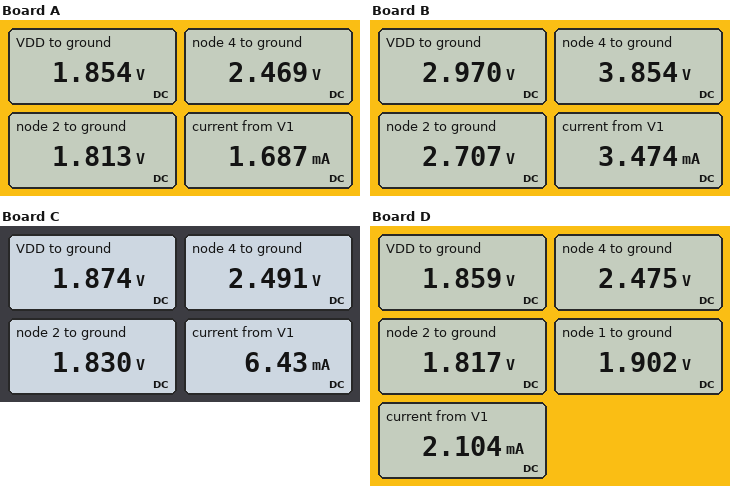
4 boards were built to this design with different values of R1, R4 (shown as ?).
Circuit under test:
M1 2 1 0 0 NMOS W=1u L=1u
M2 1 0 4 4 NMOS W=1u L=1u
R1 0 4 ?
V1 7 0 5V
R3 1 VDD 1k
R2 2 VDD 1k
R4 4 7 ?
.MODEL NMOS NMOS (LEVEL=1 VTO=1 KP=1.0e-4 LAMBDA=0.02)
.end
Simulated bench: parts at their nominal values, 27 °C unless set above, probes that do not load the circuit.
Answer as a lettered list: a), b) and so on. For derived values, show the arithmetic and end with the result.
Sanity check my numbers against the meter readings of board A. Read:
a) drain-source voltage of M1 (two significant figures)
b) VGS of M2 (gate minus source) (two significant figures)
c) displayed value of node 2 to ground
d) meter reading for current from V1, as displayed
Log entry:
a) 1.813 V = 1.8 V
b) 0 V - 2.469 V = -2.5 V
c) 1.813 V
d) 1.687 mA
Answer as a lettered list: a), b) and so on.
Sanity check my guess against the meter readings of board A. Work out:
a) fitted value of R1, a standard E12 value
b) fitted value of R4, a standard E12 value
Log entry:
a) 1.5 kΩ
b) 1.5 kΩ
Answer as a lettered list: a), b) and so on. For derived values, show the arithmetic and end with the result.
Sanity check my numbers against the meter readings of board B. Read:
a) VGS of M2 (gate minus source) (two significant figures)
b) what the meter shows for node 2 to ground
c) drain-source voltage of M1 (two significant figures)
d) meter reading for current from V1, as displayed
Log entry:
a) 0 V - 3.854 V = -3.9 V
b) 2.707 V
c) 2.707 V = 2.7 V
d) 3.474 mA
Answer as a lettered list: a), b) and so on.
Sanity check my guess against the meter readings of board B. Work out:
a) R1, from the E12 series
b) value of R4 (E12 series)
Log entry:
a) 1.2 kΩ
b) 330 Ω
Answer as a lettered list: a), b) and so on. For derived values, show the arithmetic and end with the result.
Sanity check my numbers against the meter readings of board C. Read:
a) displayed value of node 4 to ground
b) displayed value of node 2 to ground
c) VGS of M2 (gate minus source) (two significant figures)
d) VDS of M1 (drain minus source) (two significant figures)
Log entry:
a) 2.491 V
b) 1.830 V
c) 0 V - 2.491 V = -2.5 V
d) 1.83 V = 1.8 V
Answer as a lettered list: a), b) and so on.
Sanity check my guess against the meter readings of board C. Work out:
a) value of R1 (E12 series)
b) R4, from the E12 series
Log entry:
a) 390 Ω
b) 390 Ω
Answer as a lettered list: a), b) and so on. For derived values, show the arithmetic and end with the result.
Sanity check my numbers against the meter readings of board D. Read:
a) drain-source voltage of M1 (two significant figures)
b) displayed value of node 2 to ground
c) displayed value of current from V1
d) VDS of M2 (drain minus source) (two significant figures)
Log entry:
a) 1.817 V = 1.8 V
b) 1.817 V
c) 2.104 mA
d) 1.902 V - 2.475 V = -570 mV
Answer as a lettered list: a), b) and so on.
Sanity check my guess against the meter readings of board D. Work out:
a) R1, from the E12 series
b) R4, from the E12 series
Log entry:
a) 1.2 kΩ
b) 1.2 kΩ
